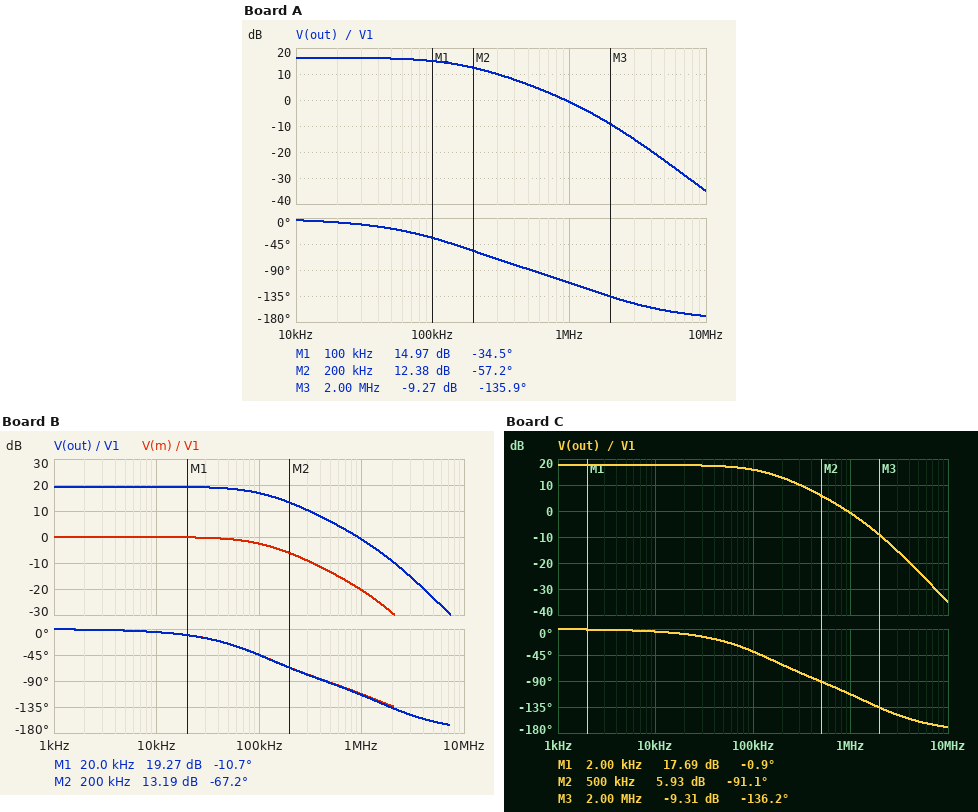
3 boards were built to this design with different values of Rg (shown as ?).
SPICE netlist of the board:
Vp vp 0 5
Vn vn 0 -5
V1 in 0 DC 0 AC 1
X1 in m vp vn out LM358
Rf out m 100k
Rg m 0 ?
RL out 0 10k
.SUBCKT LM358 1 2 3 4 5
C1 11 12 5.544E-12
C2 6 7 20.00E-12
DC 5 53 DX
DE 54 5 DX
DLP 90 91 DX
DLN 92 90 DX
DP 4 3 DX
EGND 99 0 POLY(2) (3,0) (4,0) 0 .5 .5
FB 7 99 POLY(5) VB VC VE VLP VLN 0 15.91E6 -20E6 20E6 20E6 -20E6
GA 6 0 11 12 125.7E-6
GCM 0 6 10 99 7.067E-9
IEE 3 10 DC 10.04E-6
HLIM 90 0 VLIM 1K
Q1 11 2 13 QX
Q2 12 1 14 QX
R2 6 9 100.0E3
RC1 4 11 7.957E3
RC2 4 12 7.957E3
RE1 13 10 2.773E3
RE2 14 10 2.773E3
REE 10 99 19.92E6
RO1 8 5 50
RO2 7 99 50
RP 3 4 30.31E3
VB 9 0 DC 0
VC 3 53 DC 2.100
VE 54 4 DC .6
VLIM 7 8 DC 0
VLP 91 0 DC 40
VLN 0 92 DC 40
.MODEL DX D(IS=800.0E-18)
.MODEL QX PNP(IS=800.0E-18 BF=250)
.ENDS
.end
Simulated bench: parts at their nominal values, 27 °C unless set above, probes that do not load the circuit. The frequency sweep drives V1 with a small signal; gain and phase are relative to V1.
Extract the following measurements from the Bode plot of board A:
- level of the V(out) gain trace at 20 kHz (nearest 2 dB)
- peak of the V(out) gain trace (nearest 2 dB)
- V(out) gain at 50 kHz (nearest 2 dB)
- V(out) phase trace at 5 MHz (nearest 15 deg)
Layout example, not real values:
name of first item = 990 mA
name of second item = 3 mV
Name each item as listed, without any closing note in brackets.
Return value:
level of the V(out) gain trace at 20 kHz = 16 dB
peak of the V(out) gain trace = 16 dB
V(out) gain at 50 kHz = 16 dB
V(out) phase trace at 5 MHz = -165 deg
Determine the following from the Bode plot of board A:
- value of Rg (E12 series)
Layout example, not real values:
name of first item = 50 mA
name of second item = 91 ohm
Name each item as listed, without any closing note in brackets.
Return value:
value of Rg = 18 kΩ
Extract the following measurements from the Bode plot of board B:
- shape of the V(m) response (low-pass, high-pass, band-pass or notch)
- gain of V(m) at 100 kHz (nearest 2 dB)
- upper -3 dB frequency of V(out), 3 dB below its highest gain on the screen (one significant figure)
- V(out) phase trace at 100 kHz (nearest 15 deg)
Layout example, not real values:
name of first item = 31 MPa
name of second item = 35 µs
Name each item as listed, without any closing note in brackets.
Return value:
shape of the V(m) response = low-pass
gain of V(m) at 100 kHz = -2 dB
upper -3 dB frequency of V(out), 3 dB below its highest gain on the screen = 100 kHz
V(out) phase trace at 100 kHz = -45 deg
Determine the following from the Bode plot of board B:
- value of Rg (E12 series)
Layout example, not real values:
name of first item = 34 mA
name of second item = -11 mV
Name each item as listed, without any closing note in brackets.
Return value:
value of Rg = 12 kΩ
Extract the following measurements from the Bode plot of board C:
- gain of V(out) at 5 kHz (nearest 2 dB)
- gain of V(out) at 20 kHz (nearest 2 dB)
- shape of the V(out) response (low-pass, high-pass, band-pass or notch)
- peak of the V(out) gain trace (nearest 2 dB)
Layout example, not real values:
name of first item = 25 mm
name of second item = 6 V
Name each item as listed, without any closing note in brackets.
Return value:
gain of V(out) at 5 kHz = 18 dB
gain of V(out) at 20 kHz = 18 dB
shape of the V(out) response = low-pass
peak of the V(out) gain trace = 18 dB
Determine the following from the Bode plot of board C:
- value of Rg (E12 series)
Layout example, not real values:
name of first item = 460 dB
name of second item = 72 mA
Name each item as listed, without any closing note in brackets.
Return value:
value of Rg = 15 kΩ
